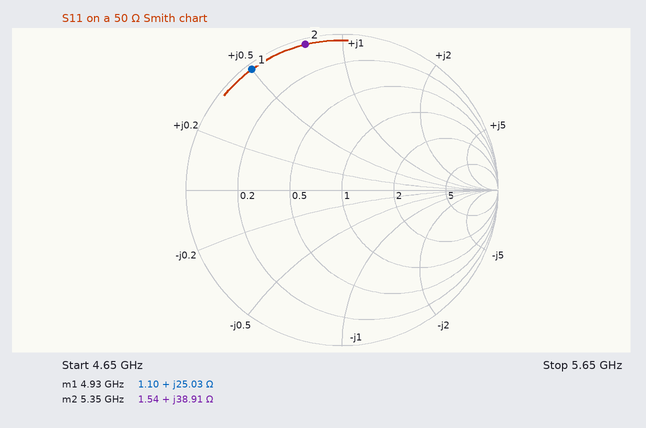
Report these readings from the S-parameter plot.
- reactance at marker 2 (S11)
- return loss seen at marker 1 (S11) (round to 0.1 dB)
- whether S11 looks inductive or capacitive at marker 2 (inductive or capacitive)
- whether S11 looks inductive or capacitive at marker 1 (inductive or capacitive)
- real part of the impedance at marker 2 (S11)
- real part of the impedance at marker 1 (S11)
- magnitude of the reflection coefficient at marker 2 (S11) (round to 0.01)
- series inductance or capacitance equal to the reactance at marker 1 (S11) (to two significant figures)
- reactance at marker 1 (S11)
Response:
+38.91 Ω
0.3 dB
inductive
inductive
1.54 Ω
1.10 Ω
0.96
810 pH
+25.03 Ω
